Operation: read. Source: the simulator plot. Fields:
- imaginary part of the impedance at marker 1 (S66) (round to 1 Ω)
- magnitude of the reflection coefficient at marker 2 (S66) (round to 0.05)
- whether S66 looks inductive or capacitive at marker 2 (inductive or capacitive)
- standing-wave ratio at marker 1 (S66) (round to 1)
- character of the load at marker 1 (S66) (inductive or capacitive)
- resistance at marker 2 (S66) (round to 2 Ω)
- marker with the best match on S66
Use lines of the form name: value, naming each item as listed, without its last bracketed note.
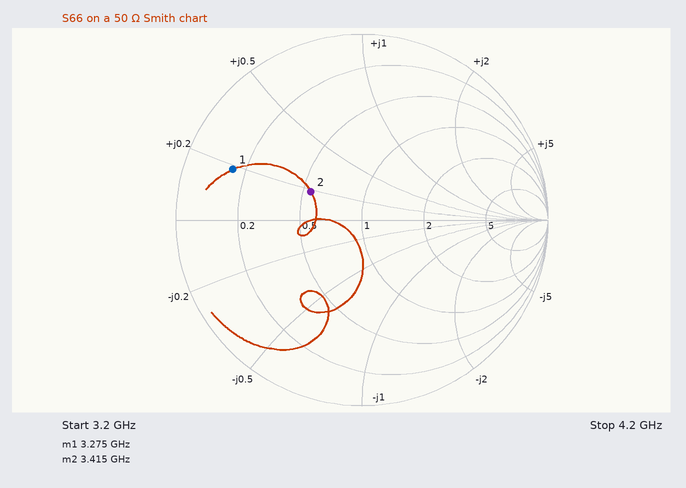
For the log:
imaginary part of the impedance at marker 1 (S66): +9 Ω
magnitude of the reflection coefficient at marker 2 (S66): 0.30
whether S66 looks inductive or capacitive at marker 2: inductive
standing-wave ratio at marker 1 (S66): 7
character of the load at marker 1 (S66): inductive
resistance at marker 2 (S66): 28 Ω
marker with the best match on S66: marker 2
